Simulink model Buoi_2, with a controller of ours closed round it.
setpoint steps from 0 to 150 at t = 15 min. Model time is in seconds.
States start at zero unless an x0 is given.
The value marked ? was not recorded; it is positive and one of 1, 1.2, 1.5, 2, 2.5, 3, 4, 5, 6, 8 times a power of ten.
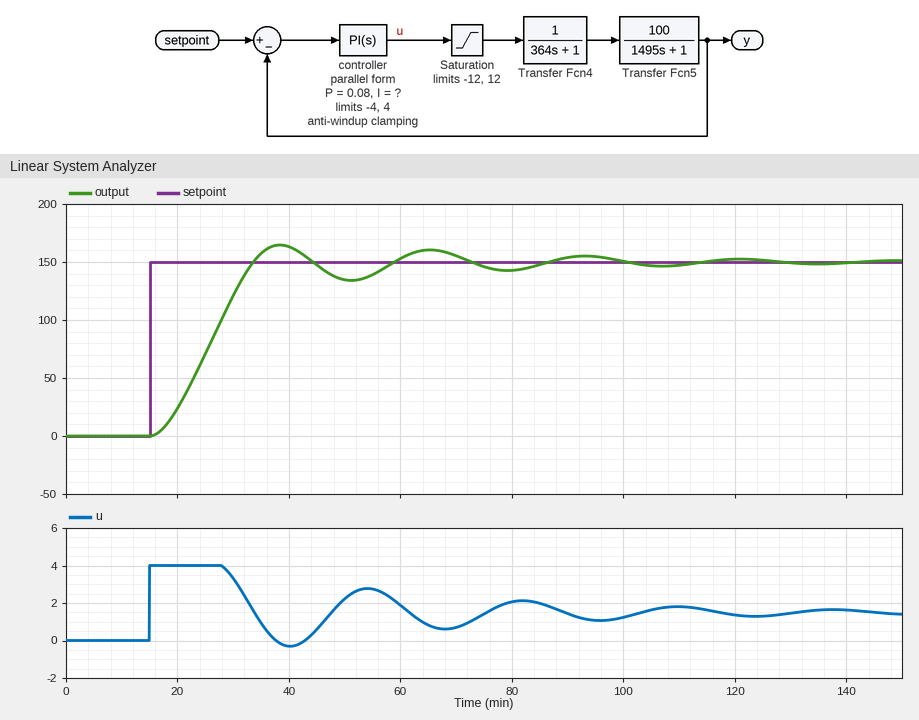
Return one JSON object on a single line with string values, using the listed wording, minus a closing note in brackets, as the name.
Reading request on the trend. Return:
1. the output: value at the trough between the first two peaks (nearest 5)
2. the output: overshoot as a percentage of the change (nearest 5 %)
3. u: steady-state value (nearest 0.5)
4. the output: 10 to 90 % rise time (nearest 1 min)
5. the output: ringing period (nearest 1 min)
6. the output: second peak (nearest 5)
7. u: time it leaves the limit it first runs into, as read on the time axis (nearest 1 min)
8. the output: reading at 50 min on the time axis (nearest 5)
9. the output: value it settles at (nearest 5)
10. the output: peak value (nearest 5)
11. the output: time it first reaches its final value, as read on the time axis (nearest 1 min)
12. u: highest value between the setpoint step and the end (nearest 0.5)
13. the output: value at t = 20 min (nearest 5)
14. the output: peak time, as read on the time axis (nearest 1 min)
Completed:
{"the output: value at the trough between the first two peaks": "135", "the output: overshoot as a percentage of the change": "10 %", "u: steady-state value": "1.5", "the output: 10 to 90 % rise time": "13 min", "the output: ringing period": "27 min", "the output: second peak": "160", "u: time it leaves the limit it first runs into, as read on the time axis": "28 min", "the output: reading at 50 min on the time axis": "135", "the output: value it settles at": "150", "the output: peak value": "165", "the output: time it first reaches its final value, as read on the time axis": "34 min", "u: highest value between the setpoint step and the end": "4.0", "the output: value at t = 20 min": "25", "the output: peak time, as read on the time axis": "38 min"}
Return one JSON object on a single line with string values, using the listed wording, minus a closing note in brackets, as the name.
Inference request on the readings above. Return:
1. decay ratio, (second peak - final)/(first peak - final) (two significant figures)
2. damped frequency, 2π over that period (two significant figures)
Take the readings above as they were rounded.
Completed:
{"decay ratio, (second peak - final)/(first peak - final)": "0.67", "damped frequency, 2π over that period": "0.23 rad/min"}
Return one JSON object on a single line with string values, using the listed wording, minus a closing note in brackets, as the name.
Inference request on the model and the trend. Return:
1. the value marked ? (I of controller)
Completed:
{"the value marked ?": "0.0002"}
